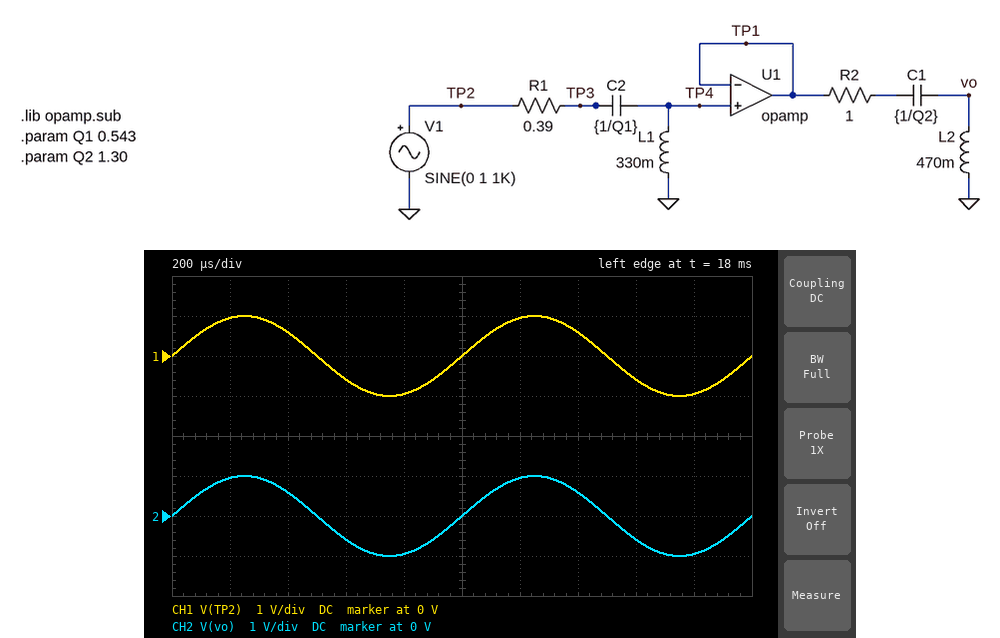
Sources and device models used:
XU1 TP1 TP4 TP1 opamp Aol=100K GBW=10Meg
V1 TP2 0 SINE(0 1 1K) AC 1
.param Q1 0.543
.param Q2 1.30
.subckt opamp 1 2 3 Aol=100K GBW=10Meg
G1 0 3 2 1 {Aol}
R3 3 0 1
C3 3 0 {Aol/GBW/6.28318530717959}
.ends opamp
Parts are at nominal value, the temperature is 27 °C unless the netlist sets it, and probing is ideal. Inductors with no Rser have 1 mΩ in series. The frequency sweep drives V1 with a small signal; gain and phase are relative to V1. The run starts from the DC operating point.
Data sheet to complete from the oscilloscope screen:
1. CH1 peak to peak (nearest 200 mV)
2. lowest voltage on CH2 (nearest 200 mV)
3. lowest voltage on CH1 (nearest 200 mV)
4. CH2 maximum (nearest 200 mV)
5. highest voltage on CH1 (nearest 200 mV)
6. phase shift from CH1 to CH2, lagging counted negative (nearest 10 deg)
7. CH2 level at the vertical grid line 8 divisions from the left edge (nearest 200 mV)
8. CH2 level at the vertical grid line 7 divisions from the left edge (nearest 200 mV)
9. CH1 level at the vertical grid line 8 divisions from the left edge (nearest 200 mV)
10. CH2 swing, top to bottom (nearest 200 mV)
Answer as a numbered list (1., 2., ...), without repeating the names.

1. 2.0 V
2. -1.0 V
3. -1.0 V
4. 1.0 V
5. 1.0 V
6. 0 deg
7. -600 mV
8. 600 mV
9. -600 mV
10. 2.0 V
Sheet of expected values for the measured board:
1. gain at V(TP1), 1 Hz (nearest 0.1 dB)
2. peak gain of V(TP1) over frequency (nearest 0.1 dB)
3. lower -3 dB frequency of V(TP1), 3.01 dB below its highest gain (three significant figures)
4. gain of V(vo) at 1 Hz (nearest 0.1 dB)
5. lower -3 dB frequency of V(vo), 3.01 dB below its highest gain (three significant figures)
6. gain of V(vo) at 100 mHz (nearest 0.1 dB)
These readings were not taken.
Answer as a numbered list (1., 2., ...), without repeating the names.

1. 0.2 dB
2. 1.7 dB
3. 173 mHz
4. 0.3 dB
5. 232 mHz
6. -28.1 dB
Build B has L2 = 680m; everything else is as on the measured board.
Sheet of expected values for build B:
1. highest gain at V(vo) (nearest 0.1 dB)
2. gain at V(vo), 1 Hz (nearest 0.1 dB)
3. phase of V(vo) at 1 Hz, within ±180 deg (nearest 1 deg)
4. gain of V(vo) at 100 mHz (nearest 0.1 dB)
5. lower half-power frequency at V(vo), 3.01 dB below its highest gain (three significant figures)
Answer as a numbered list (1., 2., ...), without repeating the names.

1. 2.5 dB
2. 0.4 dB
3. 25 deg
4. -24.4 dB
5. 205 mHz
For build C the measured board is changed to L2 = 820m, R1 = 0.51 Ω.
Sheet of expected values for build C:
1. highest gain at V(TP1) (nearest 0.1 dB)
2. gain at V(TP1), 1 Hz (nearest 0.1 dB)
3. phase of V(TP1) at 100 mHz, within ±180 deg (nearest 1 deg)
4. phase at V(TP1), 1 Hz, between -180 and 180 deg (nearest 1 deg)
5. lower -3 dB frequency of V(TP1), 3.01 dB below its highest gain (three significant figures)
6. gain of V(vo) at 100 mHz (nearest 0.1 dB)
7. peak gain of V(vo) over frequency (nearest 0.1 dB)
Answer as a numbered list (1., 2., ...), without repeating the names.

1. 0.3 dB
2. 0.1 dB
3. 142 deg
4. 14 deg
5. 184 mHz
6. -23.2 dB
7. 1.6 dB
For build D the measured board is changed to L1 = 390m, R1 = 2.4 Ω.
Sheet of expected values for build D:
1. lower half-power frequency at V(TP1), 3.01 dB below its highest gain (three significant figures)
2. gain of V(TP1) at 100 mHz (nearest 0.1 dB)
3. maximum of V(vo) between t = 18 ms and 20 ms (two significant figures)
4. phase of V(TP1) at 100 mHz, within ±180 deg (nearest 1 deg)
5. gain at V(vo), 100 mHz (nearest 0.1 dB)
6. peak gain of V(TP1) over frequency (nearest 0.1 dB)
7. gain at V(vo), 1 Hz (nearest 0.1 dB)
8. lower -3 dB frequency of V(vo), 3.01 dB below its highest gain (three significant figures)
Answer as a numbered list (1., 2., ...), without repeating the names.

1. 944 mHz
2. -20.1 dB
3. 1.0 V
4. 104 deg
5. -36.9 dB
6. 0 dB
7. -2.7 dB
8. 923 mHz
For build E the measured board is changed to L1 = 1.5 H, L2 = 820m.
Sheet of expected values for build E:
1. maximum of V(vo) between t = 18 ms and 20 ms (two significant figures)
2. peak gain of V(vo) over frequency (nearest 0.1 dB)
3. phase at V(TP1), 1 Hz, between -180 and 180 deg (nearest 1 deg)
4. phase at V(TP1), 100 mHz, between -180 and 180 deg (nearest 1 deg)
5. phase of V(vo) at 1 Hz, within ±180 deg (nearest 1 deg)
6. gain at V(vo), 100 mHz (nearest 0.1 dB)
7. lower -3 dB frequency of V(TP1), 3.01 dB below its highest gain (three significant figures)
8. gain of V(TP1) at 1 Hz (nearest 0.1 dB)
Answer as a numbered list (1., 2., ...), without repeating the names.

1. 1.0 V
2. 2.6 dB
3. 2 deg
4. 79 deg
5. 14 deg
6. -3.6 dB
7. 83.1 mHz
8. 0.1 dB
